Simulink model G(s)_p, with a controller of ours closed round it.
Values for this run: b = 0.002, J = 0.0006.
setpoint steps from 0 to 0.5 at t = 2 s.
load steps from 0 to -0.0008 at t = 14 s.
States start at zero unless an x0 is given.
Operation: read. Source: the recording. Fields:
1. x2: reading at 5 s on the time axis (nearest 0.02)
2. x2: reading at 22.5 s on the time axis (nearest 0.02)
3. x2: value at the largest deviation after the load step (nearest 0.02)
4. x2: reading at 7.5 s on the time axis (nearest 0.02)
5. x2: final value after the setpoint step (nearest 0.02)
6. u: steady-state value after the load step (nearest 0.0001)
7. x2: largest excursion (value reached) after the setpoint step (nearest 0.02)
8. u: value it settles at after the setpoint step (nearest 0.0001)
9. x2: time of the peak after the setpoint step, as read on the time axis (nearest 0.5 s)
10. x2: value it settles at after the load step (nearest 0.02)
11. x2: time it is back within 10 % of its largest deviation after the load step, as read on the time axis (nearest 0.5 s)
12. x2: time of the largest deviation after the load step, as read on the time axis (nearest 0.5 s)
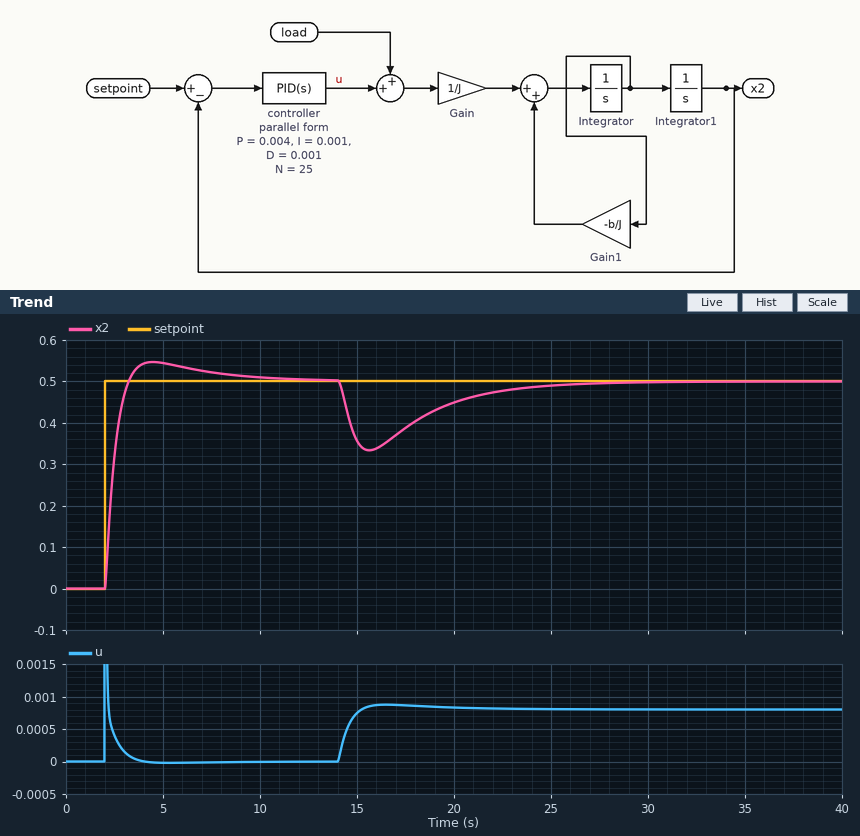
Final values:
0.54
0.48
0.34
0.52
0.50
0.0008
0.54
0.0000
4.5 s
0.50
23.5 s
15.5 s
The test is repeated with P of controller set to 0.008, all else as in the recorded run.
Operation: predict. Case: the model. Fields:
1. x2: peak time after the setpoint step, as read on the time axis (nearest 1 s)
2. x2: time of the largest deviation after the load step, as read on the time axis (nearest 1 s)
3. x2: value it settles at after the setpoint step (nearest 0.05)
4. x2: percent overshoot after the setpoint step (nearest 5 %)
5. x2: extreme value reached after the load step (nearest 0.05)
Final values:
3 s
15 s
0.50
10 %
0.40
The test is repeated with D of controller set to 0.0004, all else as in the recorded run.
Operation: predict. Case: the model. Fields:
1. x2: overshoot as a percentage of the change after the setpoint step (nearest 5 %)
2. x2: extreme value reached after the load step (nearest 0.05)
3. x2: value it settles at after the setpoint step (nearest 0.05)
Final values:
15 %
0.30
0.50
